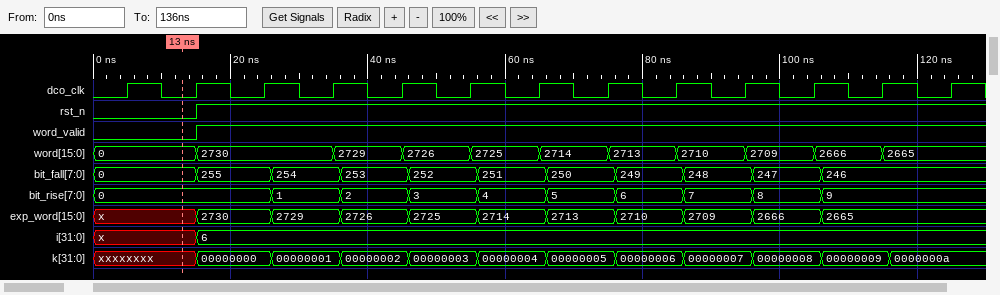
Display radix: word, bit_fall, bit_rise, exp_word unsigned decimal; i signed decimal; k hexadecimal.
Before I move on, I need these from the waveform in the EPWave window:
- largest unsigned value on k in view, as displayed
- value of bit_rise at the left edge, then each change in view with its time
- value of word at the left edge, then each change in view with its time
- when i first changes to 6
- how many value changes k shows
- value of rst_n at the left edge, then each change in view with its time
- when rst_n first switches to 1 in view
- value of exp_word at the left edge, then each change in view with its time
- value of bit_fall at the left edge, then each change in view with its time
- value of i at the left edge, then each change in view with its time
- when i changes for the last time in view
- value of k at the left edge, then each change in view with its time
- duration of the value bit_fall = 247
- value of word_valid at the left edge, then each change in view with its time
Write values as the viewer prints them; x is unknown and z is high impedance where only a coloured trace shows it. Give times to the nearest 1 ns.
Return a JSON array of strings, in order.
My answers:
["0000000a", "0, 1 at 26 ns, 2 at 36 ns, 3 at 46 ns, 4 at 56 ns, 5 at 66 ns, 6 at 76 ns, 7 at 86 ns, 8 at 96 ns, 9 at 106 ns", "0, 2730 at 15 ns, 2729 at 35 ns, 2726 at 45 ns, 2725 at 55 ns, 2714 at 65 ns, 2713 at 75 ns, 2710 at 85 ns, 2709 at 95 ns, 2666 at 105 ns, 2665 at 115 ns", "15 ns", "11", "0, 1 at 15 ns", "15 ns", "x, 2730 at 15 ns, 2729 at 26 ns, 2726 at 36 ns, 2725 at 46 ns, 2714 at 56 ns, 2713 at 66 ns, 2710 at 76 ns, 2709 at 86 ns, 2666 at 96 ns, 2665 at 106 ns", "0, 255 at 15 ns, 254 at 26 ns, 253 at 36 ns, 252 at 46 ns, 251 at 56 ns, 250 at 66 ns, 249 at 76 ns, 248 at 86 ns, 247 at 96 ns, 246 at 106 ns", "x, 6 at 15 ns", "15 ns", "xxxxxxxx, 00000000 at 15 ns, 00000001 at 26 ns, 00000002 at 36 ns, 00000003 at 46 ns, 00000004 at 56 ns, 00000005 at 66 ns, 00000006 at 76 ns, 00000007 at 86 ns, 00000008 at 96 ns, 00000009 at 106 ns, 0000000a at 116 ns", "10 ns", "0, 1 at 15 ns"]
